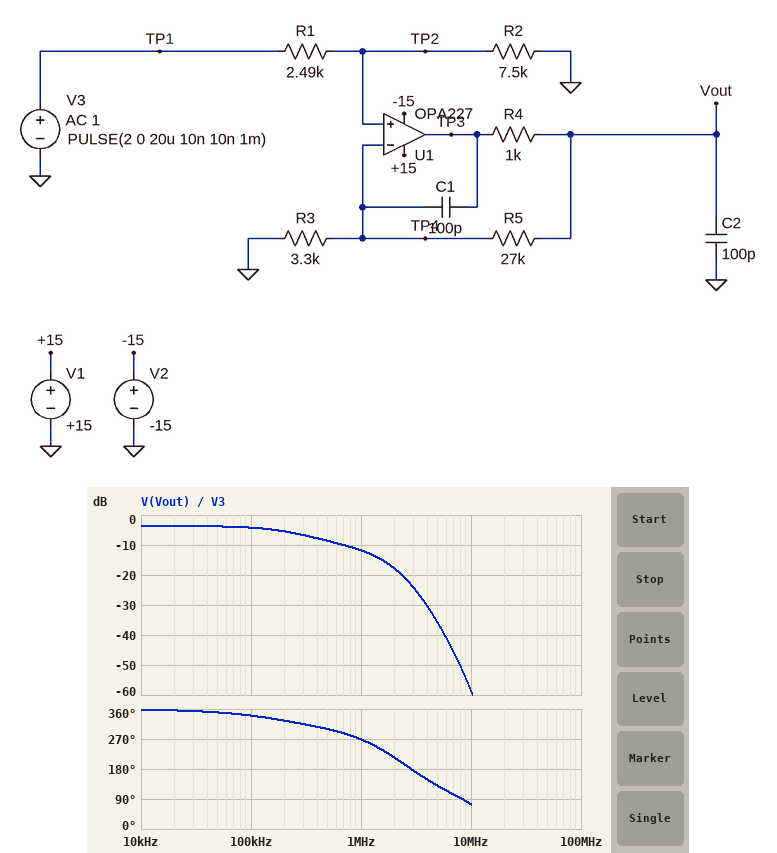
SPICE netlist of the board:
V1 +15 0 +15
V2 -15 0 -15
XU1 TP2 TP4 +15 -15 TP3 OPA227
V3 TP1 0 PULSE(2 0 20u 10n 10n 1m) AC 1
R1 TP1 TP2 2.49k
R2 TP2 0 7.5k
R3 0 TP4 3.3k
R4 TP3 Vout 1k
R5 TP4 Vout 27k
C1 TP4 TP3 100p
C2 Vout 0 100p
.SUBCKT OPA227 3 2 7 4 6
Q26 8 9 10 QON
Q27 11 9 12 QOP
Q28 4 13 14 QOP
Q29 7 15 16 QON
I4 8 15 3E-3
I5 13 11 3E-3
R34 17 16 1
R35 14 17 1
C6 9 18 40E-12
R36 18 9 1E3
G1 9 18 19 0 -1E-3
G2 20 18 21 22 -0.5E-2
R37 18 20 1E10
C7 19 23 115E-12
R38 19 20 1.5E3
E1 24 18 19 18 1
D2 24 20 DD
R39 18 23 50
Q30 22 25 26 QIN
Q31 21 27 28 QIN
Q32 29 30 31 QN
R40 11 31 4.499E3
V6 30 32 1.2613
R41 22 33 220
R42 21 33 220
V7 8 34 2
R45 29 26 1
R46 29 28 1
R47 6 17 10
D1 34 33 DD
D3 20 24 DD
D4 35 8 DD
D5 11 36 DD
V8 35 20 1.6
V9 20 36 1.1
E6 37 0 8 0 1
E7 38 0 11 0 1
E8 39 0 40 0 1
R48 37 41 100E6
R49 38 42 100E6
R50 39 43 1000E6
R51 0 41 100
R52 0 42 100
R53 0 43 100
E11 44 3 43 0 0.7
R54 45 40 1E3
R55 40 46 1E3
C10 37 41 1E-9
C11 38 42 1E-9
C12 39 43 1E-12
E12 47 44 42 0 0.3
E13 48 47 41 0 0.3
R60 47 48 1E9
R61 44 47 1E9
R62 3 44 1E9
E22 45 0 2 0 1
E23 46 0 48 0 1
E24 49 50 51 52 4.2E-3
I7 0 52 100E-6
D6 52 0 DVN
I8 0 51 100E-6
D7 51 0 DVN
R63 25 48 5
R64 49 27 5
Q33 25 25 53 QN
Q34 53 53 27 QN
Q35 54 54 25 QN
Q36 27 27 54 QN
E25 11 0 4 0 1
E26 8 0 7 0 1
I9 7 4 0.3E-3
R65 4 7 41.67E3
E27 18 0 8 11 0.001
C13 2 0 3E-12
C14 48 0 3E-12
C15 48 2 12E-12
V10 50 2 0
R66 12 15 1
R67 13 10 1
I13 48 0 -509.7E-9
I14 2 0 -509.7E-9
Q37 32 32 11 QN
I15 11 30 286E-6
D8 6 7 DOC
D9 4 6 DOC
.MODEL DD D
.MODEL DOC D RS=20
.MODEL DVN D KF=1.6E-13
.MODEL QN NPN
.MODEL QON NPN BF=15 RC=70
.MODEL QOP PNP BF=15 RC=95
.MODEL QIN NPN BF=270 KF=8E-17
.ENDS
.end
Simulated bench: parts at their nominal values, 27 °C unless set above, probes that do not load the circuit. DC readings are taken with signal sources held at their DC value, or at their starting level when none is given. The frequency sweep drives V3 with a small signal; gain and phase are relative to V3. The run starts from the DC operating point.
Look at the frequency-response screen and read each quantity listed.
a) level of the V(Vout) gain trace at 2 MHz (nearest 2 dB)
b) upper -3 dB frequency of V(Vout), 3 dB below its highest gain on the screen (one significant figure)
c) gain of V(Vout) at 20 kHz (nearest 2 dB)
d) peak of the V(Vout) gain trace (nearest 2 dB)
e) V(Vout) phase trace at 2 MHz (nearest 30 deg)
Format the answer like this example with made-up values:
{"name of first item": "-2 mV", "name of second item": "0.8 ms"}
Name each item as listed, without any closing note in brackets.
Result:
{"level of the V(Vout) gain trace at 2 MHz": "-18 dB", "upper -3 dB frequency of V(Vout), 3 dB below its highest gain on the screen": "300 kHz", "gain of V(Vout) at 20 kHz": "-4 dB", "peak of the V(Vout) gain trace": "-4 dB", "V(Vout) phase trace at 2 MHz": "210 deg"}
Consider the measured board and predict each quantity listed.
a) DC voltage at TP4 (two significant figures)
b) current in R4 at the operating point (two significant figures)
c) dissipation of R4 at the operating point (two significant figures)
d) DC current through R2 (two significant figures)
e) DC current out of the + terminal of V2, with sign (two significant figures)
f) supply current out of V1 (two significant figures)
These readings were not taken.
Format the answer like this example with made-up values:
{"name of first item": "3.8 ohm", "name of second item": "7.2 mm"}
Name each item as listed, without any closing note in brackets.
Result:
{"DC voltage at TP4": "1.5 V", "current in R4 at the operating point": "450 µA", "dissipation of R4 at the operating point": "200 µW", "DC current through R2": "200 µA", "DC current out of the + terminal of V2, with sign": "-3.5 mA", "supply current out of V1": "3.9 mA"}
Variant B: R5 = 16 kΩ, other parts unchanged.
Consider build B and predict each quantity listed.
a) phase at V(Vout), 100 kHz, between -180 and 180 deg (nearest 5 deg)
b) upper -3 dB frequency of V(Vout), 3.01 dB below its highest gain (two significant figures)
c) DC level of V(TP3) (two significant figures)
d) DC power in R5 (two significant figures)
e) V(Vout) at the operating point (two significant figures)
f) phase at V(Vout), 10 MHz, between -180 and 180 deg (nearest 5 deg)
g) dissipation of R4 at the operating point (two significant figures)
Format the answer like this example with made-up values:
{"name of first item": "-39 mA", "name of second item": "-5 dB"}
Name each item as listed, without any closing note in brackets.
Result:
{"phase at V(Vout), 100 kHz, between -180 and 180 deg": "-40 deg", "upper -3 dB frequency of V(Vout), 3.01 dB below its highest gain": "96 kHz", "DC level of V(TP3)": "9.2 V", "DC power in R5": "3.3 mW", "V(Vout) at the operating point": "8.8 V", "phase at V(Vout), 10 MHz, between -180 and 180 deg": "85 deg", "dissipation of R4 at the operating point": "210 µW"}
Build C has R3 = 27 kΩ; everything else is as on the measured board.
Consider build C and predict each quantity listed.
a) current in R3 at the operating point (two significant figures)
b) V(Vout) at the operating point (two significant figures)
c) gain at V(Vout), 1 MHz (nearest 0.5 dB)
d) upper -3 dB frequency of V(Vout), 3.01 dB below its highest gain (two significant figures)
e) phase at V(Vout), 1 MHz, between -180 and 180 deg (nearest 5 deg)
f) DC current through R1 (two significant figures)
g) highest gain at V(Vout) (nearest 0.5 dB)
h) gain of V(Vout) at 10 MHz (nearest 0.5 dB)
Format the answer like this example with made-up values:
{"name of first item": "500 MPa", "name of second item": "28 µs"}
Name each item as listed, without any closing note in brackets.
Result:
{"current in R3 at the operating point": "56 µA", "V(Vout) at the operating point": "3.0 V", "gain at V(Vout), 1 MHz": "-3.0 dB", "upper -3 dB frequency of V(Vout), 3.01 dB below its highest gain": "88 kHz", "phase at V(Vout), 1 MHz, between -180 and 180 deg": "-45 deg", "DC current through R1": "200 µA", "highest gain at V(Vout)": "3.5 dB", "gain of V(Vout) at 10 MHz": "-34.0 dB"}
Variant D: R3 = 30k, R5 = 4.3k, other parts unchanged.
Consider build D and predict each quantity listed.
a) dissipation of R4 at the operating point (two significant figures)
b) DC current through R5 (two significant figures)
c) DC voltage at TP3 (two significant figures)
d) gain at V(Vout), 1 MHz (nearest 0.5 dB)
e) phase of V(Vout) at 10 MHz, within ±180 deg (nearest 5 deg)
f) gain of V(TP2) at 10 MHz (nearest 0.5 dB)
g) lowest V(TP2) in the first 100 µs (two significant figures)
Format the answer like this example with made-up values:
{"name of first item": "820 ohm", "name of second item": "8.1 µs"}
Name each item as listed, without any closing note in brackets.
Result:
{"dissipation of R4 at the operating point": "2.5 µW", "DC current through R5": "50 µA", "DC voltage at TP3": "1.8 V", "gain at V(Vout), 1 MHz": "-1.5 dB", "phase of V(Vout) at 10 MHz, within ±180 deg": "85 deg", "gain of V(TP2) at 10 MHz": "-8.5 dB", "lowest V(TP2) in the first 100 µs": "-44 mV"}
